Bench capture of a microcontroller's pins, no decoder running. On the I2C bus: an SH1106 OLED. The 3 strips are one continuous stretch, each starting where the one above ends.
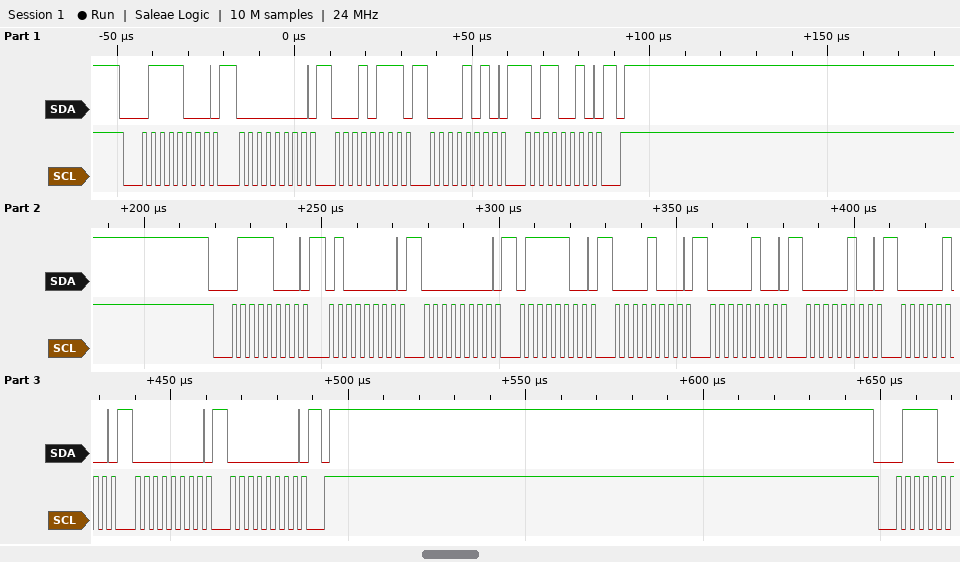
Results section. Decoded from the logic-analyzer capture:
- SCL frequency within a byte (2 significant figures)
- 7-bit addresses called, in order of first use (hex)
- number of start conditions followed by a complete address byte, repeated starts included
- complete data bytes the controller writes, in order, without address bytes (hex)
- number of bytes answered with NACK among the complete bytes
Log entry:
400 kHz
0x3C
2
00 17 0A B2 40 00 7C 08 04 04 04 00 00
0
